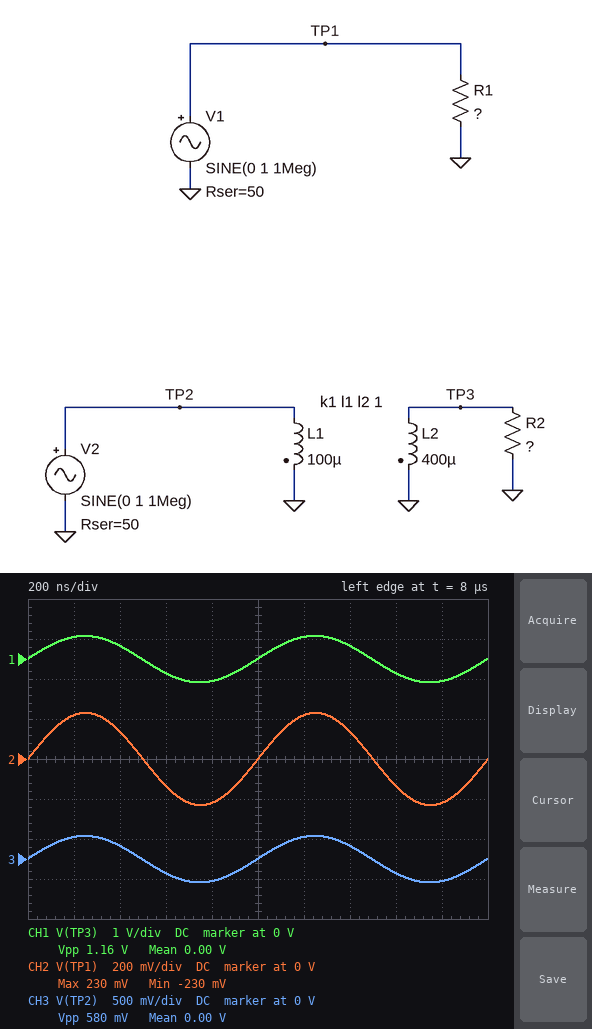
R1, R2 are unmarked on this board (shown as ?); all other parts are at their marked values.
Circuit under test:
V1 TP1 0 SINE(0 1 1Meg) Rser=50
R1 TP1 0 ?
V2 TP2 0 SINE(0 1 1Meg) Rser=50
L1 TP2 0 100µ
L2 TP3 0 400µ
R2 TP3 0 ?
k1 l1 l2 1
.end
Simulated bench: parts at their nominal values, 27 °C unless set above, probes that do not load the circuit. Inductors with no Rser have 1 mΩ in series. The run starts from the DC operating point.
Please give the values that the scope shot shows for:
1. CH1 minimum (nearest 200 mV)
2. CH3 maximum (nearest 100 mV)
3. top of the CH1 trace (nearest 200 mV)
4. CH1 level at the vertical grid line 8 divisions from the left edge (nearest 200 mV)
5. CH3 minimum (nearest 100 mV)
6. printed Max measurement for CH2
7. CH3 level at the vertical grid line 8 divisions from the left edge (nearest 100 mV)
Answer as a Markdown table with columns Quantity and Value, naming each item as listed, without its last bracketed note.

| Quantity | Value |
|---|---|
| CH1 minimum | -600 mV |
| CH3 maximum | 300 mV |
| top of the CH1 trace | 600 mV |
| CH1 level at the vertical grid line 8 divisions from the left edge | -400 mV |
| CH3 minimum | -300 mV |
| printed Max measurement for CH2 | 230 mV |
| CH3 level at the vertical grid line 8 divisions from the left edge | -200 mV |
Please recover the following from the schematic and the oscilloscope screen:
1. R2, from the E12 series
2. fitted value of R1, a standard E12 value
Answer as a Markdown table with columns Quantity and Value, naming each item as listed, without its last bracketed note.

| Quantity | Value |
|---|---|
| R2, from the E12 series | 82 Ω |
| fitted value of R1, a standard E12 value | 15 Ω |
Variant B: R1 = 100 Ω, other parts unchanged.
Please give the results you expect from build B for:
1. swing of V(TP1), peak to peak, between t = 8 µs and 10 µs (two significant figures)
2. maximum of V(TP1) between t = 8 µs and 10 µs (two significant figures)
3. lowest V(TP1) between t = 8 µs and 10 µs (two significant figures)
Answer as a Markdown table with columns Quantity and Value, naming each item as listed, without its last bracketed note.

| Quantity | Value |
|---|---|
| swing of V(TP1), peak to peak, between t = 8 µs and 10 µs | 1.3 V |
| maximum of V(TP1) between t = 8 µs and 10 µs | 670 mV |
| lowest V(TP1) between t = 8 µs and 10 µs | -670 mV |
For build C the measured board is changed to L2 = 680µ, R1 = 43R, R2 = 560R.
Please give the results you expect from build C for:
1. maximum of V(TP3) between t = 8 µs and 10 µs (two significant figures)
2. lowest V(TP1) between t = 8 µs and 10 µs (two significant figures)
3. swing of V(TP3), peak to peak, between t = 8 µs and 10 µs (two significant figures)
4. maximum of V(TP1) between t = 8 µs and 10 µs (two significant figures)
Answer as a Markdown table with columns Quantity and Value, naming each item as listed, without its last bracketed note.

| Quantity | Value |
|---|---|
| maximum of V(TP3) between t = 8 µs and 10 µs | 1.6 V |
| lowest V(TP1) between t = 8 µs and 10 µs | -460 mV |
| swing of V(TP3), peak to peak, between t = 8 µs and 10 µs | 3.2 V |
| maximum of V(TP1) between t = 8 µs and 10 µs | 460 mV |
